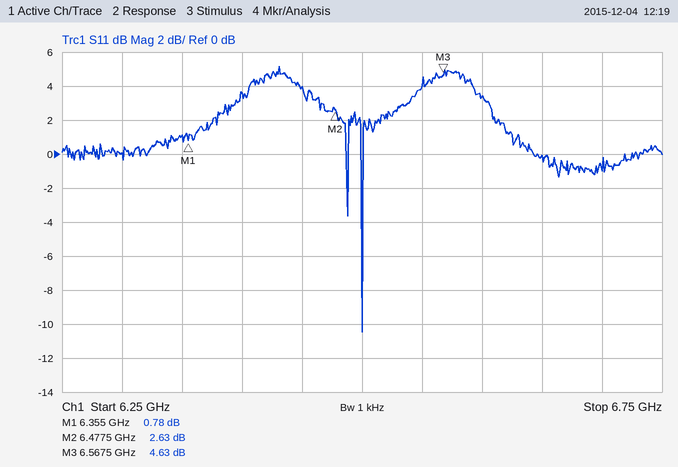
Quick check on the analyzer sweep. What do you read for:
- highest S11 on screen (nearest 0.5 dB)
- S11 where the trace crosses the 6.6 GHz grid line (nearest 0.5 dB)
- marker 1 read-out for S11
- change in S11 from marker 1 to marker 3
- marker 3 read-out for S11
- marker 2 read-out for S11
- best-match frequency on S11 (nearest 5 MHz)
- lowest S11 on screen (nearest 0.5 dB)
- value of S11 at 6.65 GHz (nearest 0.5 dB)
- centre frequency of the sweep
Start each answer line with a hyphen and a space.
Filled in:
- 5.0 dB
- 3.5 dB
- 0.78 dB
- 3.85 dB
- 4.63 dB
- 2.63 dB
- 6.500 GHz
- -10.5 dB
- 0.0 dB
- 6.5 GHz
